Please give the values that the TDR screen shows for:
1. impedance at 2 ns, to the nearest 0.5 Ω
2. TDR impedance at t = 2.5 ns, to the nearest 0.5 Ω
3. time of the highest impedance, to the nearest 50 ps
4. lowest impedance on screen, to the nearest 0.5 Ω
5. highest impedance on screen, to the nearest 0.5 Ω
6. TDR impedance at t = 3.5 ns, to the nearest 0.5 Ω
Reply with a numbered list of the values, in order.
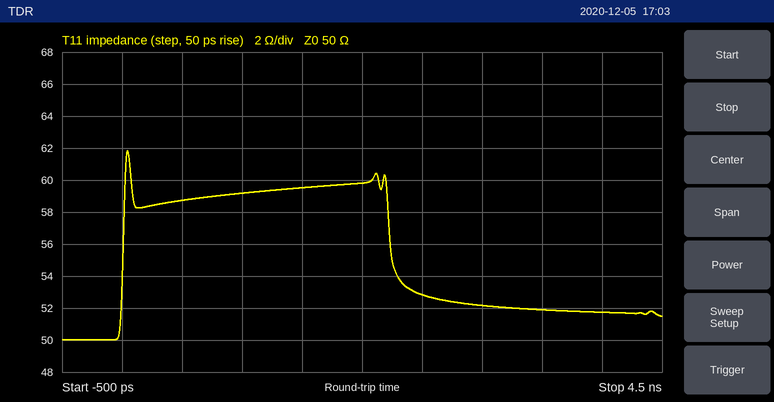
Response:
1. 60.0 Ω
2. 53.0 Ω
3. 50 ps
4. 50.0 Ω
5. 62.0 Ω
6. 52.0 Ω
